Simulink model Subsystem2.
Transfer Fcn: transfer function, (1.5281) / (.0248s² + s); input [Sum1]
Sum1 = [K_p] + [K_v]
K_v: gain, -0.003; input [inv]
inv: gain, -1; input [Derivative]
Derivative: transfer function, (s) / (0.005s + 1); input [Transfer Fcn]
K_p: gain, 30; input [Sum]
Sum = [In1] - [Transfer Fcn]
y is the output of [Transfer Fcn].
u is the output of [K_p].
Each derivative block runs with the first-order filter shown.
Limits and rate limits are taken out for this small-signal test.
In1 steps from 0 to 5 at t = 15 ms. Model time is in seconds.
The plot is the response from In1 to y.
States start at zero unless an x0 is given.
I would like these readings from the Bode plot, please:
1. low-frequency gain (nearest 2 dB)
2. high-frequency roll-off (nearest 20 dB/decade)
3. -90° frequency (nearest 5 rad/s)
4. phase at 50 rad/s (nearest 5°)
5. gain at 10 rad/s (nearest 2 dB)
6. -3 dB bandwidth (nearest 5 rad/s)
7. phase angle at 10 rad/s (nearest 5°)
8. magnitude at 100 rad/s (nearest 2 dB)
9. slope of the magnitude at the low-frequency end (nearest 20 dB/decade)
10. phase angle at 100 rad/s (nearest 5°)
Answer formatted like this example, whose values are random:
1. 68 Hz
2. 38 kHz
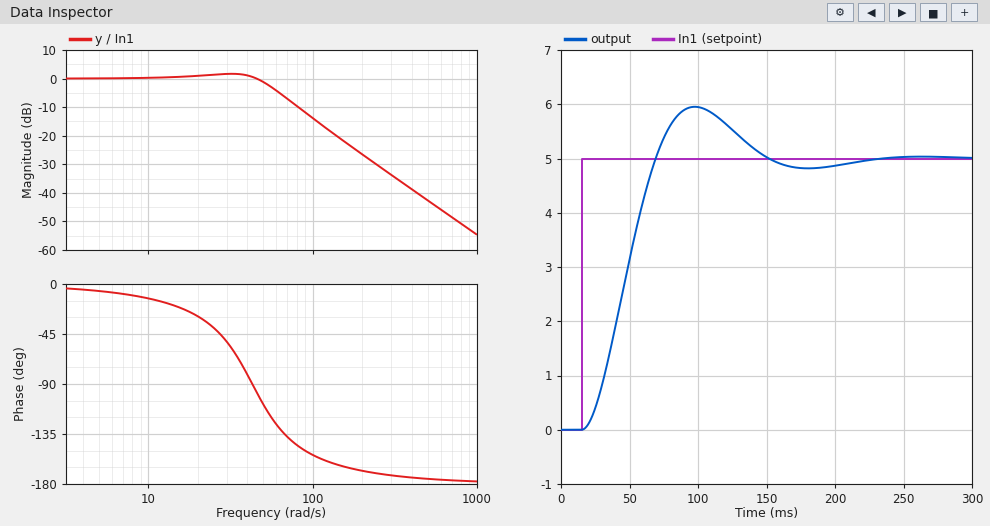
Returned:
1. 0 dB
2. -40 dB/decade
3. 45 rad/s
4. -110°
5. 0 dB
6. 55 rad/s
7. -15°
8. -14 dB
9. 0 dB/decade
10. -155°
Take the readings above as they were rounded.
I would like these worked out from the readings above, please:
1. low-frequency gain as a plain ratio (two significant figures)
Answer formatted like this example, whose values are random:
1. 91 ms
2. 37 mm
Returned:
1. 1.0
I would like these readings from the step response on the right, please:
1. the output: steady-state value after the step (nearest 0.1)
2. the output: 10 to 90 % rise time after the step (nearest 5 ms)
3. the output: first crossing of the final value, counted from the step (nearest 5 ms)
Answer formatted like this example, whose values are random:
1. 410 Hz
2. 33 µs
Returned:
1. 5.0
2. 35 ms
3. 55 ms
